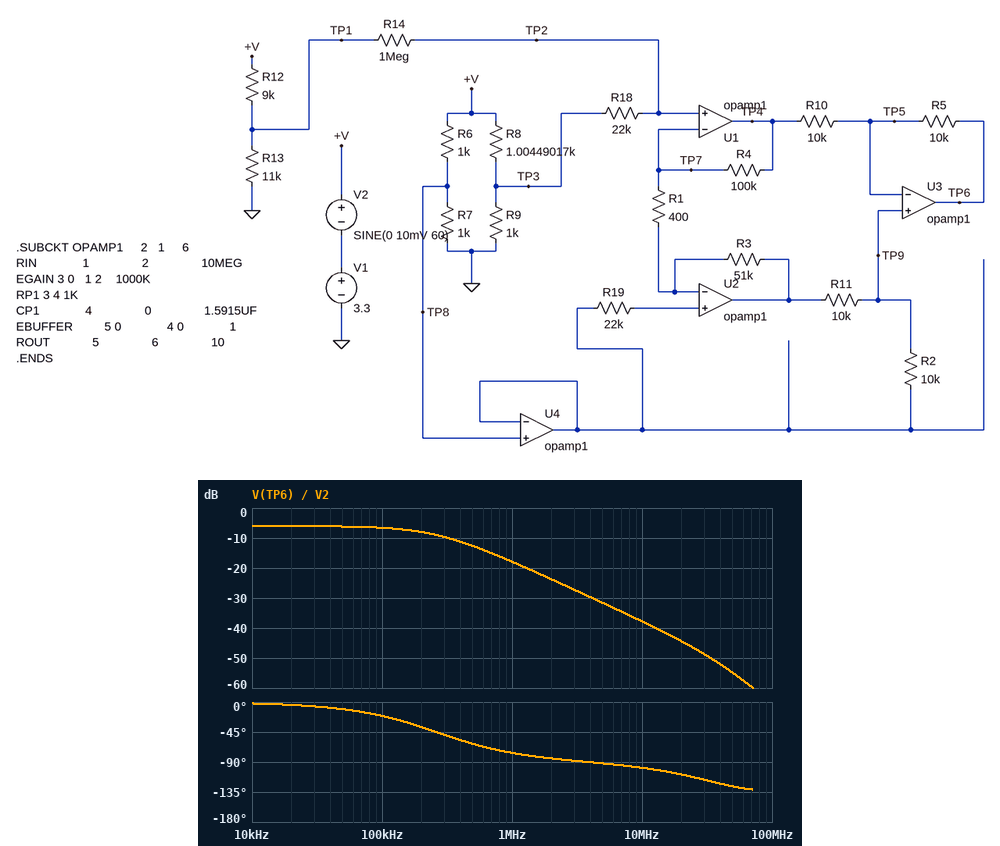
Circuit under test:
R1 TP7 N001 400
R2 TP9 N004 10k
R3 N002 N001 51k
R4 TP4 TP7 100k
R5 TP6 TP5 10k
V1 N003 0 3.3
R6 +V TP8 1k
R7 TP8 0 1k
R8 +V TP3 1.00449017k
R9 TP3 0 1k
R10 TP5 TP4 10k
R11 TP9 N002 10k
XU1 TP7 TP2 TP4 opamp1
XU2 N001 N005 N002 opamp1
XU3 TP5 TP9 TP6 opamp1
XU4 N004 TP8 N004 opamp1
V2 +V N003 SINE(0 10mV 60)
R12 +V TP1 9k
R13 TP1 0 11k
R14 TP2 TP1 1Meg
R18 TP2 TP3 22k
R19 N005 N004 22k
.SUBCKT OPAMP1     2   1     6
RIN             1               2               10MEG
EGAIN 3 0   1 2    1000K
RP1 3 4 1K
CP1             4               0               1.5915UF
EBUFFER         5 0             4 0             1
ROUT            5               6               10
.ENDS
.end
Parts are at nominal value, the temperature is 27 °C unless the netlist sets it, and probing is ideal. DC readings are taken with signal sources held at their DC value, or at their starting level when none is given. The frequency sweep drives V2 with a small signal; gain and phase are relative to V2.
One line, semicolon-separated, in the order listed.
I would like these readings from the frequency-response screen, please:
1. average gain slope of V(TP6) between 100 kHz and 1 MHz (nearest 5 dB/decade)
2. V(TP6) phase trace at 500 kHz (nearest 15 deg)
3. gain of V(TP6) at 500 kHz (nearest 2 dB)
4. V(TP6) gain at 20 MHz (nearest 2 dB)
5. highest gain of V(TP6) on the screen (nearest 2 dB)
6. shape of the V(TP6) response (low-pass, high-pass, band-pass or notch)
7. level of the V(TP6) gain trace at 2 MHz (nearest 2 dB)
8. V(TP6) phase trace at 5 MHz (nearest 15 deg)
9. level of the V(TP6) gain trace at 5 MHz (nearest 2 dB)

-10 dB/decade; -60 deg; -12 dB; -44 dB; -6 dB; low-pass; -24 dB; -90 deg; -32 dB
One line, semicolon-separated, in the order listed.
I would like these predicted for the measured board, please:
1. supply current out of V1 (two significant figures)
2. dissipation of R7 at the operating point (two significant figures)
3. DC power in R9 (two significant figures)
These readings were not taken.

3.5 mA; 2.7 mW; 2.7 mW
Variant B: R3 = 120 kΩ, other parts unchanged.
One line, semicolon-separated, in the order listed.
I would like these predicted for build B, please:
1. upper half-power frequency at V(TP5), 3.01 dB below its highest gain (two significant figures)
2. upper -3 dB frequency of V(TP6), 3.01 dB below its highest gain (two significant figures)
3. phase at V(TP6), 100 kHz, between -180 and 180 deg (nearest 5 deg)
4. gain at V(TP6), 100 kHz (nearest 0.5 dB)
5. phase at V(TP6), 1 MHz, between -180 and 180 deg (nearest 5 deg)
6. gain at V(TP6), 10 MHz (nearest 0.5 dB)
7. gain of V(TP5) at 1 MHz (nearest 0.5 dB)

19 MHz; 180 kHz; -30 deg; -7.0 dB; -80 deg; -41.0 dB; -8.5 dB
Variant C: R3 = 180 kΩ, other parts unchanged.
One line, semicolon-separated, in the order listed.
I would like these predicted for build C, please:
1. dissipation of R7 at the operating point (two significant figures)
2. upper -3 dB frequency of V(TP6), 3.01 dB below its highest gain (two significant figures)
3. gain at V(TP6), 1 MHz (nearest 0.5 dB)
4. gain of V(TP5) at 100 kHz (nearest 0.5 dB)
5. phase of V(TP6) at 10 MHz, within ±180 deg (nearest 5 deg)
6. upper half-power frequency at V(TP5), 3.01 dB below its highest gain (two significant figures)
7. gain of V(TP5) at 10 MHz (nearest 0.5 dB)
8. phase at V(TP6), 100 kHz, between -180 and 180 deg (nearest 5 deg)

2.7 mW; 140 kHz; -23.0 dB; -7.0 dB; -95 deg; 500 kHz; -9.5 dB; -35 deg
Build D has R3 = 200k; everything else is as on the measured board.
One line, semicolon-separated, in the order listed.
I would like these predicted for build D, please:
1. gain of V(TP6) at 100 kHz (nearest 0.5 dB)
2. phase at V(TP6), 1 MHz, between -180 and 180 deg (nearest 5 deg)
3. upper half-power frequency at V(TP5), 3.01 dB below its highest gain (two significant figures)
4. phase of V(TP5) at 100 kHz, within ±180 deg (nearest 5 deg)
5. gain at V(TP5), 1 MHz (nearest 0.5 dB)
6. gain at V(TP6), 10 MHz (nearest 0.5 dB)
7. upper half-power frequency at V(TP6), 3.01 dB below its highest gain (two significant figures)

-8.0 dB; -85 deg; 400 kHz; -10 deg; -9.5 dB; -43.5 dB; 130 kHz
